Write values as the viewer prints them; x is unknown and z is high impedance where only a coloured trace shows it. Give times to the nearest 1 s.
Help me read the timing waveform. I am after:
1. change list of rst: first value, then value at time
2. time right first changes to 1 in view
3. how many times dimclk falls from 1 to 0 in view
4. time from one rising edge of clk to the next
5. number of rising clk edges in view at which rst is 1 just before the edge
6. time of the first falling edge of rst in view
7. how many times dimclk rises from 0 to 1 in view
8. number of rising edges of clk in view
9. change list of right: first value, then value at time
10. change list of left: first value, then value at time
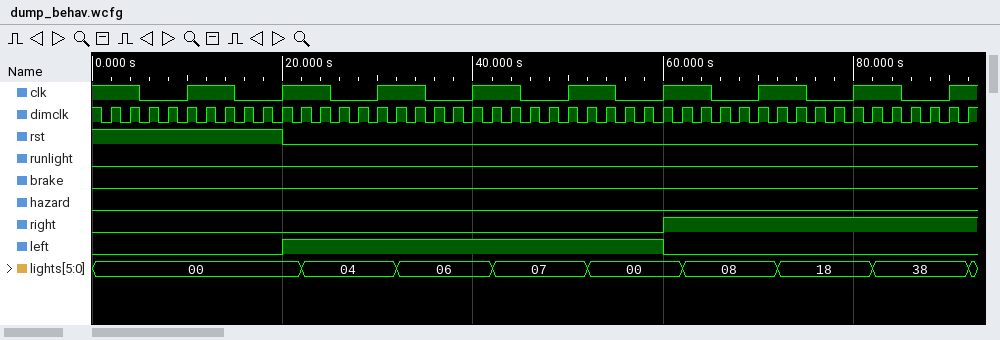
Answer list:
1, 0 at 20 s
60 s
46
10 s
2
20 s
46
9
0, 1 at 60 s
0, 1 at 20 s, 0 at 60 s
